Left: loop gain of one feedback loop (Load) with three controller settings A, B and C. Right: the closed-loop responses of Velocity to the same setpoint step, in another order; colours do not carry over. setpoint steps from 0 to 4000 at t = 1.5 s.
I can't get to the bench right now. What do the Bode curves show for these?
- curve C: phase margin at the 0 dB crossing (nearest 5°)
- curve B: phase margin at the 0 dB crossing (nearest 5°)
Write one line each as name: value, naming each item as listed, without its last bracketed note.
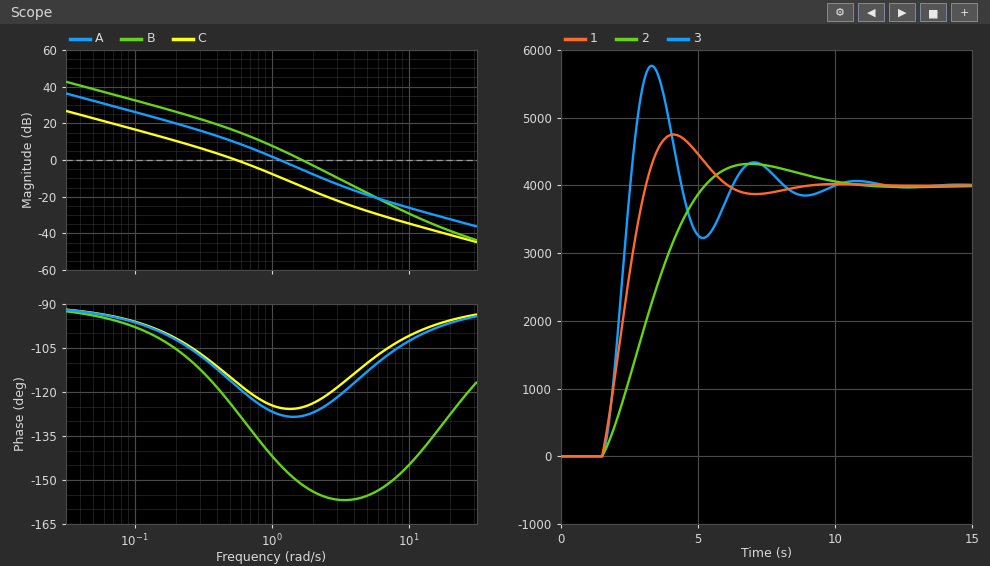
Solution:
curve C: phase margin at the 0 dB crossing: 65°
curve B: phase margin at the 0 dB crossing: 30°
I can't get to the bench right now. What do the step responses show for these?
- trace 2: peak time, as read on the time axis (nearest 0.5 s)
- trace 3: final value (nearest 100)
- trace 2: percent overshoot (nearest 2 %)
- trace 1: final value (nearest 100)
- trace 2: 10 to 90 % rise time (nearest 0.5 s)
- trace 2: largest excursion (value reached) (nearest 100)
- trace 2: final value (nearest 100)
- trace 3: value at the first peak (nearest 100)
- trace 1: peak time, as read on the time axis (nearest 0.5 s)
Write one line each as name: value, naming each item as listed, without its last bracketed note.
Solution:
trace 2: peak time, as read on the time axis: 7.0 s
trace 3: final value: 4000
trace 2: percent overshoot: 8 %
trace 1: final value: 4000
trace 2: 10 to 90 % rise time: 2.5 s
trace 2: largest excursion (value reached): 4300
trace 2: final value: 4000
trace 3: value at the first peak: 5800
trace 1: peak time, as read on the time axis: 4.0 s
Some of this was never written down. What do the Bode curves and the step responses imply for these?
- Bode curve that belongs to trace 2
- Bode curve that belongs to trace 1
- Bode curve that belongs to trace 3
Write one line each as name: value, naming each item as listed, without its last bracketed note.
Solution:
Bode curve that belongs to trace 2: C
Bode curve that belongs to trace 1: A
Bode curve that belongs to trace 3: B
